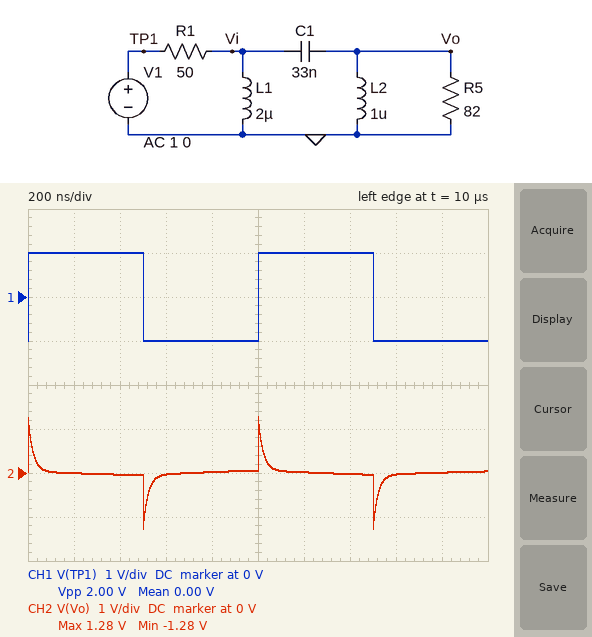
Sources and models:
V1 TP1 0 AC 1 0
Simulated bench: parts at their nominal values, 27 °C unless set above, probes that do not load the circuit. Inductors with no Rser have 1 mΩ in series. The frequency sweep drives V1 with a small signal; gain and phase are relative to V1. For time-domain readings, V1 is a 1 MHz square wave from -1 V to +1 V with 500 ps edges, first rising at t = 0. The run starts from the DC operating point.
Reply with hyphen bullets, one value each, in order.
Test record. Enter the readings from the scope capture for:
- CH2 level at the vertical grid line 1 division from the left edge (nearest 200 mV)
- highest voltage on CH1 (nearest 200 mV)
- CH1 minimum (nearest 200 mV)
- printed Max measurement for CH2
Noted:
- 0 V
- 1.0 V
- -1.0 V
- 1.28 V
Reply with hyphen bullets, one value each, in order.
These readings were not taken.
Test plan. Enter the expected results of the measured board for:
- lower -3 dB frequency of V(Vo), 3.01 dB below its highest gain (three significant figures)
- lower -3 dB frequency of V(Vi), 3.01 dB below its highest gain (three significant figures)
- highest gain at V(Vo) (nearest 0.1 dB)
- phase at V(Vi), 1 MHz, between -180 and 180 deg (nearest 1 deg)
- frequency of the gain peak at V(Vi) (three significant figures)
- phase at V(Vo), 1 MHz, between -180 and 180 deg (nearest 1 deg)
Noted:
- 7.33 MHz
- 480 kHz
- -4.1 dB
- 72 deg
- 505 kHz
- 86 deg
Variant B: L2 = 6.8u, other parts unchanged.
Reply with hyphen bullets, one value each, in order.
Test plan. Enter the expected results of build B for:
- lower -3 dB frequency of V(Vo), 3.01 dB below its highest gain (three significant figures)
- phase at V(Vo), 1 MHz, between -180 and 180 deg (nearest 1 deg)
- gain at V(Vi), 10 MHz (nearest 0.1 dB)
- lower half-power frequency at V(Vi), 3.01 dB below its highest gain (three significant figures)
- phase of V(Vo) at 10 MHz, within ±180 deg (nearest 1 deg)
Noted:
- 3.14 MHz
- 75 deg
- -4.6 dB
- 3.21 MHz
- 18 deg
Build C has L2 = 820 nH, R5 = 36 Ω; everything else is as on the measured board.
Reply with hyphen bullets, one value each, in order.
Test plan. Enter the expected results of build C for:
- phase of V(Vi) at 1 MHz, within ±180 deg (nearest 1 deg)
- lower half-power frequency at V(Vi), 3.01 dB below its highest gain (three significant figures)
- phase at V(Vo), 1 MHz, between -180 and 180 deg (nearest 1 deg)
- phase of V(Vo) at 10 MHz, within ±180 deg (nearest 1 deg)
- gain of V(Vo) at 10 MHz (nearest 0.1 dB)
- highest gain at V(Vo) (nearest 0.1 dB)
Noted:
- 20 deg
- 490 kHz
- 85 deg
- 30 deg
- -8.8 dB
- -7.6 dB
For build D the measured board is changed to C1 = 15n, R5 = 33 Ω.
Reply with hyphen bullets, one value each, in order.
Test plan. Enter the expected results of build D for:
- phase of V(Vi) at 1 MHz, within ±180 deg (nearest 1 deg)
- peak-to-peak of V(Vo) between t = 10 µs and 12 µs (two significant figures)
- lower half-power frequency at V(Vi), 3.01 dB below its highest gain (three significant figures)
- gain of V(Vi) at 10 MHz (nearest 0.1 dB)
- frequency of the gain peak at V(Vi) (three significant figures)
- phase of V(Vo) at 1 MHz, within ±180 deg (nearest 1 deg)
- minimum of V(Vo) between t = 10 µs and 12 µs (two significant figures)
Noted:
- -60 deg
- 1.9 V
- 679 kHz
- -9.0 dB
- 745 kHz
- 95 deg
- -930 mV
